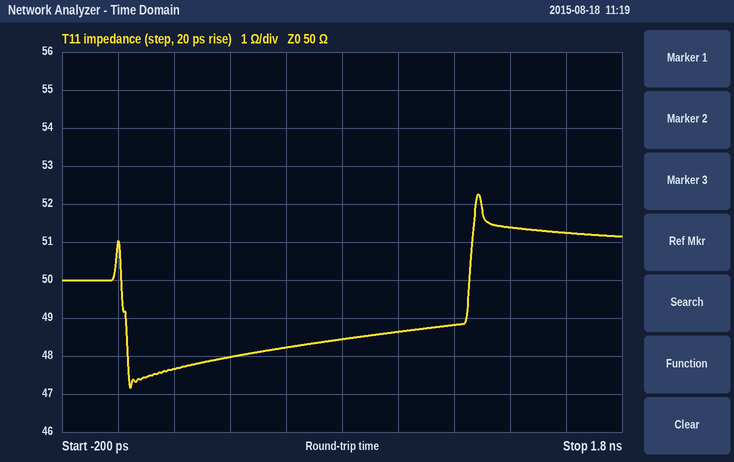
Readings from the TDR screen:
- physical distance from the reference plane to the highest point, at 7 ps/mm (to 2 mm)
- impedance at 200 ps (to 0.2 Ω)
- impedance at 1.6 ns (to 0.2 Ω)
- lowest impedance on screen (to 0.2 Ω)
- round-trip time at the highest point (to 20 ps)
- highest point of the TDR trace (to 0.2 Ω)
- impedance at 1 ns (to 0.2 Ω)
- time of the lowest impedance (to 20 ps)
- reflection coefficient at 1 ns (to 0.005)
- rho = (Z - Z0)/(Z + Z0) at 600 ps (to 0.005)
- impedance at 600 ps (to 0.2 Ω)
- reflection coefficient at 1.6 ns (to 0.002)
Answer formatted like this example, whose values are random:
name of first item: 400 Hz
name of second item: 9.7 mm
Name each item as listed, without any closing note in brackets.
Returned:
physical distance from the reference plane to the highest point, at 7 ps/mm: 92 mm
impedance at 200 ps: 47.6 Ω
impedance at 1.6 ns: 51.2 Ω
lowest impedance on screen: 47.2 Ω
round-trip time at the highest point: 1.28 ns
highest point of the TDR trace: 52.2 Ω
impedance at 1 ns: 48.6 Ω
time of the lowest impedance: 40 ps
reflection coefficient at 1 ns: -0.015
rho = (Z - Z0)/(Z + Z0) at 600 ps: -0.020
impedance at 600 ps: 48.2 Ω
reflection coefficient at 1.6 ns: +0.012
